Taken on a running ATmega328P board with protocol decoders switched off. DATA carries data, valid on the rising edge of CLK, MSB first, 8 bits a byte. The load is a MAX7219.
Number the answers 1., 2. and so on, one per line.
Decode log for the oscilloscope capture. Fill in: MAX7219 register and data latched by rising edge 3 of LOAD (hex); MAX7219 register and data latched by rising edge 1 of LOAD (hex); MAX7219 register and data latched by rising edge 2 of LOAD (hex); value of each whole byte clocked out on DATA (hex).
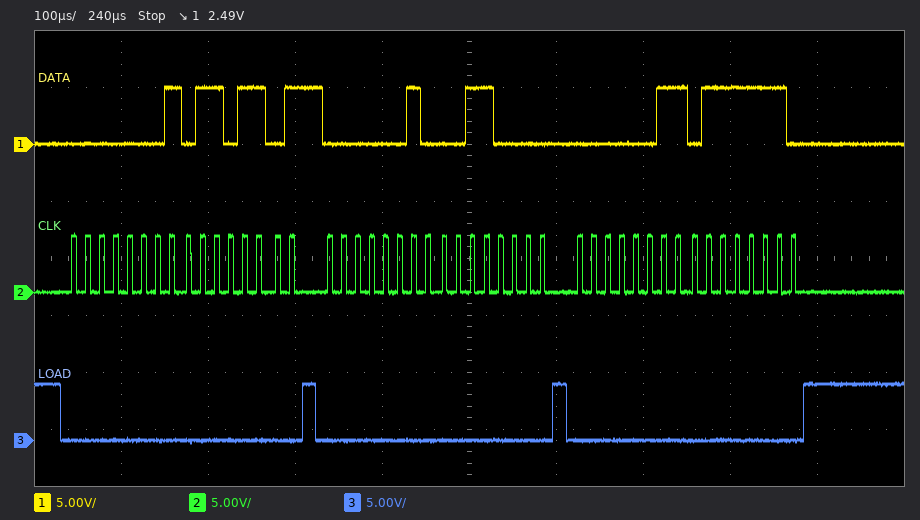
1. register 0x3, data 0x7E
2. register 0x1, data 0x6D
3. register 0x2, data 0x30
4. 01 6D 02 30 03 7E
